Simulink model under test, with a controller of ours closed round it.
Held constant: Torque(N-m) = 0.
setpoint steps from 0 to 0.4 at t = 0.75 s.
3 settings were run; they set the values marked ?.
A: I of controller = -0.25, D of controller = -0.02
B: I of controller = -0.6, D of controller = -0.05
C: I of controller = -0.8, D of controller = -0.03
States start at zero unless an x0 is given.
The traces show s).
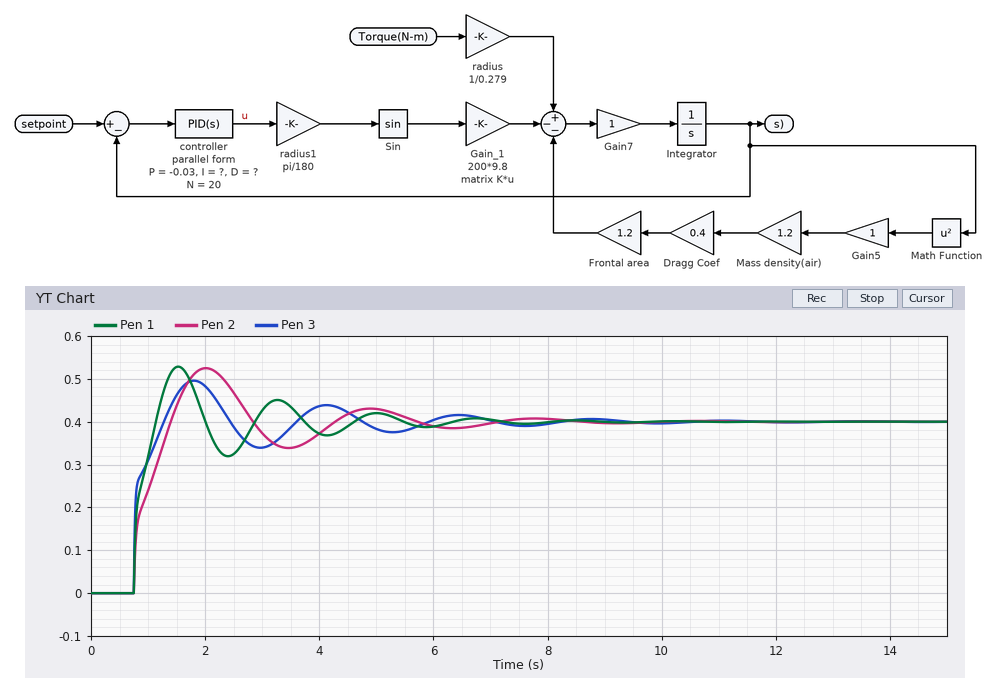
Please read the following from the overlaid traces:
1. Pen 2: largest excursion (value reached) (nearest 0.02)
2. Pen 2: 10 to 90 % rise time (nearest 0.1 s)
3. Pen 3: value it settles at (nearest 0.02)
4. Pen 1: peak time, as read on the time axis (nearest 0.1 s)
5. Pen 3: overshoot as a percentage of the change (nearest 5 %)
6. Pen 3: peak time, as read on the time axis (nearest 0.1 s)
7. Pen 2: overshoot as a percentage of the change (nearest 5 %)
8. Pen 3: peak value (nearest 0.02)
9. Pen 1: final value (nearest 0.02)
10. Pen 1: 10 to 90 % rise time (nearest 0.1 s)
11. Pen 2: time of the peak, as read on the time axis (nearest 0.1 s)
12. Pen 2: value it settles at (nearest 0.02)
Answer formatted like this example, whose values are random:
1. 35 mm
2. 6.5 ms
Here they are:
1. 0.52
2. 0.5 s
3. 0.40
4. 1.5 s
5. 25 %
6. 1.8 s
7. 30 %
8. 0.50
9. 0.40
10. 0.3 s
11. 2.0 s
12. 0.40
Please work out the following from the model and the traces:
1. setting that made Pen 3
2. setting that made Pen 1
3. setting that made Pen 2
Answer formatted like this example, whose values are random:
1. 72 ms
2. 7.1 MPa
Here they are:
1. B
2. C
3. A
